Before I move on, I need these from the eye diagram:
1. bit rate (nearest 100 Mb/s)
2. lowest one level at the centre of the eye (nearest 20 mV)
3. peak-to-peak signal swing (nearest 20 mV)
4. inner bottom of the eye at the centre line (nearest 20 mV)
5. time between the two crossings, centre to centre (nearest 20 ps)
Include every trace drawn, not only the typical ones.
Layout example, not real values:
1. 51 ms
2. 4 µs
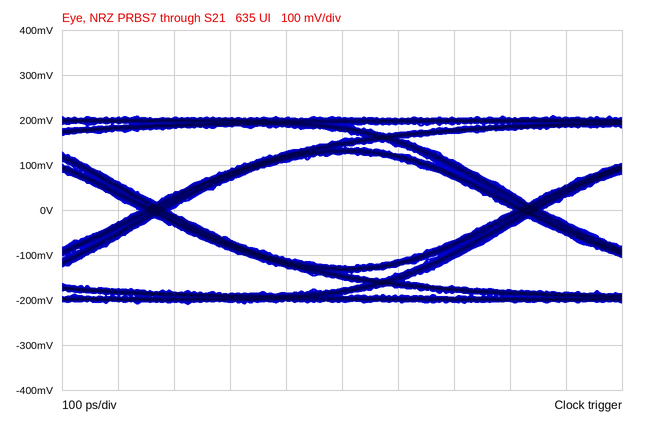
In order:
1. 1.5 Gb/s
2. 120 mV
3. 420 mV
4. -120 mV
5. 660 ps
